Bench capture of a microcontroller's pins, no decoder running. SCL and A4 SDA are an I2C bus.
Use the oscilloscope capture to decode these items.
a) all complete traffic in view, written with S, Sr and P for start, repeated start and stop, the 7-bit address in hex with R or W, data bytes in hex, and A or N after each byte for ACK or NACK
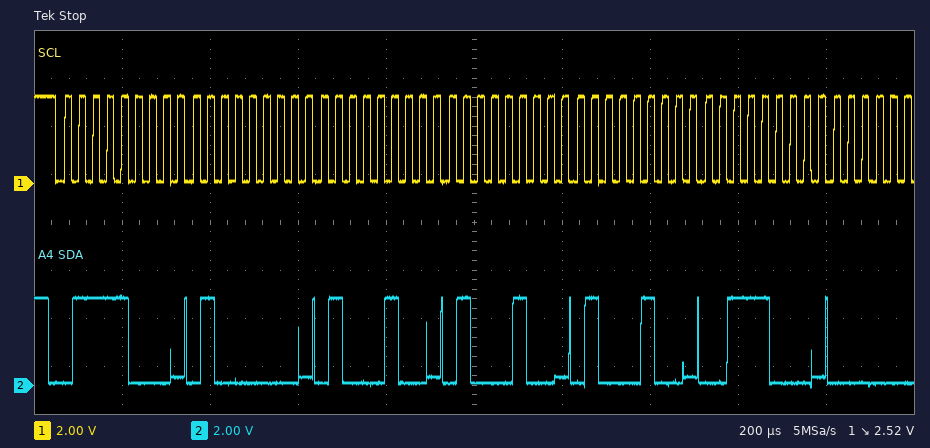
S 3CW A 40 A 44 A 44 A 44 A 38 A
